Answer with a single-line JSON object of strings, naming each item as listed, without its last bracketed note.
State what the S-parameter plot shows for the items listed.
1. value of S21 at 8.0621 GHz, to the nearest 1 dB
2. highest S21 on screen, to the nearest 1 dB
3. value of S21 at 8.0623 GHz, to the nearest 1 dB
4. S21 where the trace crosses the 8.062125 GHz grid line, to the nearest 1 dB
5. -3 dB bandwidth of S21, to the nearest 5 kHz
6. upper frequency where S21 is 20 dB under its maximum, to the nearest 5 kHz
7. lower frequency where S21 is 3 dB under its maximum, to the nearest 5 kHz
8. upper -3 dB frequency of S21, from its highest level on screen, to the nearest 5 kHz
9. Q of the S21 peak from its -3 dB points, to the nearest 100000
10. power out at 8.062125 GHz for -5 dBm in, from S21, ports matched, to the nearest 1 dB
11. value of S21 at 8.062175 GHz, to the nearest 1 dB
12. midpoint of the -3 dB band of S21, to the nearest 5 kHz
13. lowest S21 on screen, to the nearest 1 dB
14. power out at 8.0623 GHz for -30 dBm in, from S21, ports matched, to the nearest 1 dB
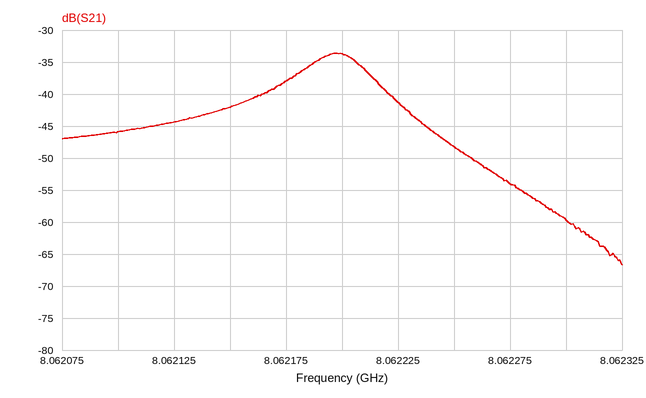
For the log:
{"value of S21 at 8.0621 GHz, to the nearest 1 dB": "-46 dB", "highest S21 on screen, to the nearest 1 dB": "-34 dB", "value of S21 at 8.0623 GHz, to the nearest 1 dB": "-60 dB", "S21 where the trace crosses the 8.062125 GHz grid line, to the nearest 1 dB": "-44 dB", "-3 dB bandwidth of S21, to the nearest 5 kHz": "30 kHz", "upper frequency where S21 is 20 dB under its maximum, to the nearest 5 kHz": "8.062275 GHz", "lower frequency where S21 is 3 dB under its maximum, to the nearest 5 kHz": "8.062180 GHz", "upper -3 dB frequency of S21, from its highest level on screen, to the nearest 5 kHz": "8.062210 GHz", "Q of the S21 peak from its -3 dB points, to the nearest 100000": "300000", "power out at 8.062125 GHz for -5 dBm in, from S21, ports matched, to the nearest 1 dB": "-49 dBm", "value of S21 at 8.062175 GHz, to the nearest 1 dB": "-38 dB", "midpoint of the -3 dB band of S21, to the nearest 5 kHz": "8.062195 GHz", "lowest S21 on screen, to the nearest 1 dB": "-67 dB", "power out at 8.0623 GHz for -30 dBm in, from S21, ports matched, to the nearest 1 dB": "-90 dBm"}
